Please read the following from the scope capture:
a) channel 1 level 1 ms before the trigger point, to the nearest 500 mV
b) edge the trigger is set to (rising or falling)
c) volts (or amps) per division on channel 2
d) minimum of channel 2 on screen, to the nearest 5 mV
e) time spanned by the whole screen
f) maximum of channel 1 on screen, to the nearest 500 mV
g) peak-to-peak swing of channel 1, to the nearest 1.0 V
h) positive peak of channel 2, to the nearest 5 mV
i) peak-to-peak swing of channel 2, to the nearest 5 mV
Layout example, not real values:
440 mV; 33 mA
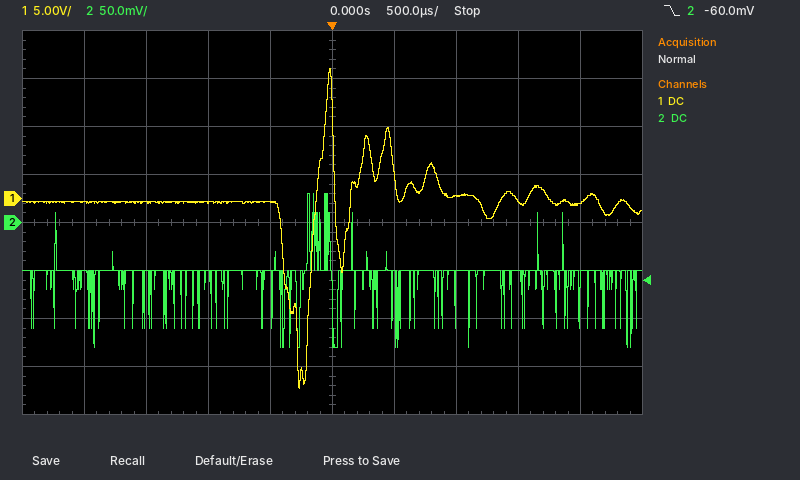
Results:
-500 mV; falling; 50 mV; -130 mV; 5 ms; 13.5 V; 33.0 V; 30 mV; 160 mV
